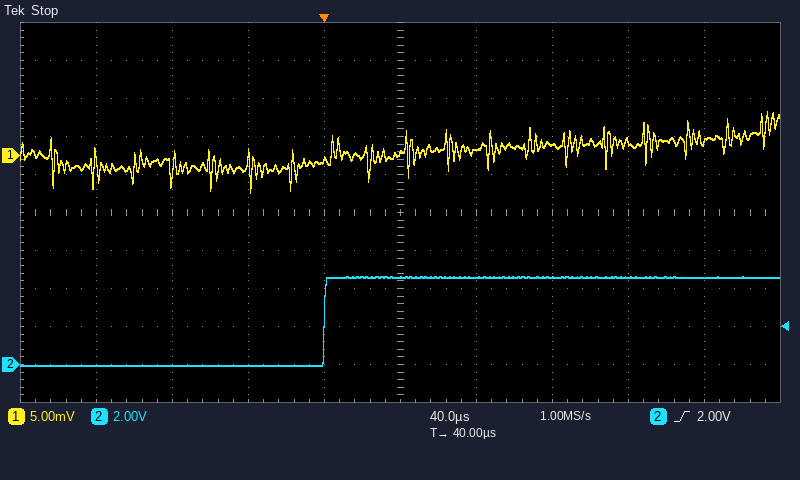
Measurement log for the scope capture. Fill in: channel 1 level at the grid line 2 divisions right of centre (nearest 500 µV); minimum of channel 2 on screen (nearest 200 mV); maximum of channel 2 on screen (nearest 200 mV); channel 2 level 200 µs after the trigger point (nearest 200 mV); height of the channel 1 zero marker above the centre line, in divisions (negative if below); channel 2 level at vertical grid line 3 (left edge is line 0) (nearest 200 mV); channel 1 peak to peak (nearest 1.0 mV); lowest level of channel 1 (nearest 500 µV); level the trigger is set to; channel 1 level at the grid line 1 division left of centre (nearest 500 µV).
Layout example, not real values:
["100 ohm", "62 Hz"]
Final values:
["1.5 mV", "0.0 V", "4.6 V", "4.6 V", "+1.5 div", "0.0 V", "11.0 mV", "-5.0 mV", "2.00 V", "-500 µV"]
